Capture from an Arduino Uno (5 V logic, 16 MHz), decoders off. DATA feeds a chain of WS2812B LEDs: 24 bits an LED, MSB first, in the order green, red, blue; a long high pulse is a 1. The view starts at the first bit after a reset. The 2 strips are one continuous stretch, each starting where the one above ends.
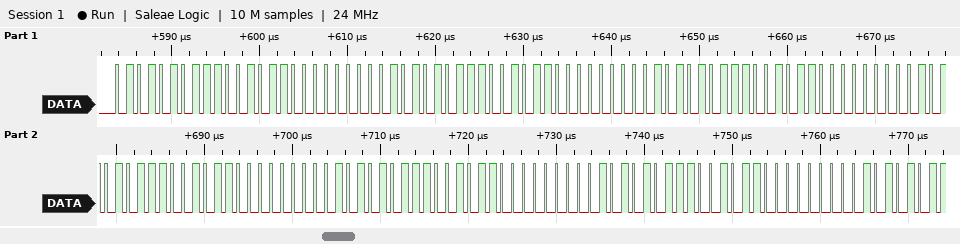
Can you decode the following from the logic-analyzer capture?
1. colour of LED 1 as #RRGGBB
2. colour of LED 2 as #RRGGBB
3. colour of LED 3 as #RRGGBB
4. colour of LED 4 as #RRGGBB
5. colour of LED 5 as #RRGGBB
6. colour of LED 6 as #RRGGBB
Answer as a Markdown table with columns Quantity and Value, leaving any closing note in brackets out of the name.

| Quantity | Value |
|---|---|
| colour of LED 1 as #RRGGBB | #CB5500 |
| colour of LED 2 as #RRGGBB | #CB5500 |
| colour of LED 3 as #RRGGBB | #CB5500 |
| colour of LED 4 as #RRGGBB | #CB5500 |
| colour of LED 5 as #RRGGBB | #CB5500 |
| colour of LED 6 as #RRGGBB | #CB5500 |
